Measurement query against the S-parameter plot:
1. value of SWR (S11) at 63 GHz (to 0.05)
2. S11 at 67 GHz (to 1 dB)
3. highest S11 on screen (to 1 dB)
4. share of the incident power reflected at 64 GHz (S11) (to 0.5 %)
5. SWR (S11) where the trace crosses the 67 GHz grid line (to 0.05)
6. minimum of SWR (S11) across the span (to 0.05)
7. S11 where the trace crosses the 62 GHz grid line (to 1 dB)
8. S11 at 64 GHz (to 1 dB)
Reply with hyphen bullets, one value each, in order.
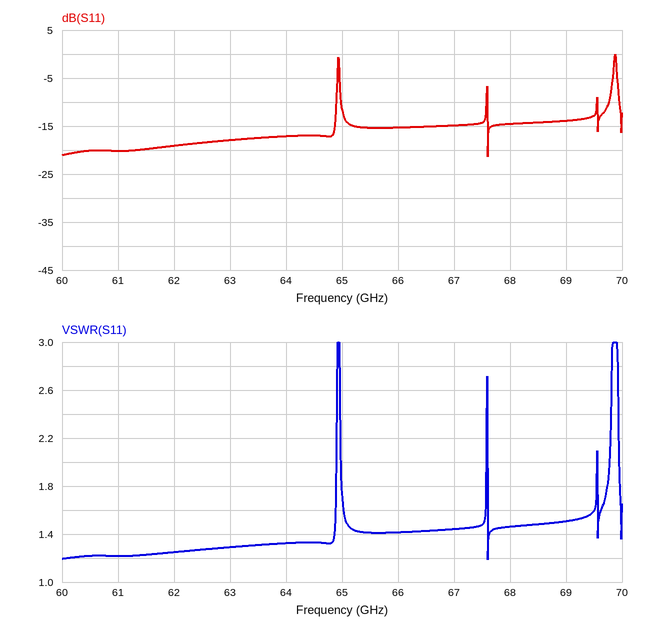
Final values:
- 1.30
- -15 dB
- 0 dB
- 2.0 %
- 1.45
- 1.20
- -19 dB
- -17 dB
